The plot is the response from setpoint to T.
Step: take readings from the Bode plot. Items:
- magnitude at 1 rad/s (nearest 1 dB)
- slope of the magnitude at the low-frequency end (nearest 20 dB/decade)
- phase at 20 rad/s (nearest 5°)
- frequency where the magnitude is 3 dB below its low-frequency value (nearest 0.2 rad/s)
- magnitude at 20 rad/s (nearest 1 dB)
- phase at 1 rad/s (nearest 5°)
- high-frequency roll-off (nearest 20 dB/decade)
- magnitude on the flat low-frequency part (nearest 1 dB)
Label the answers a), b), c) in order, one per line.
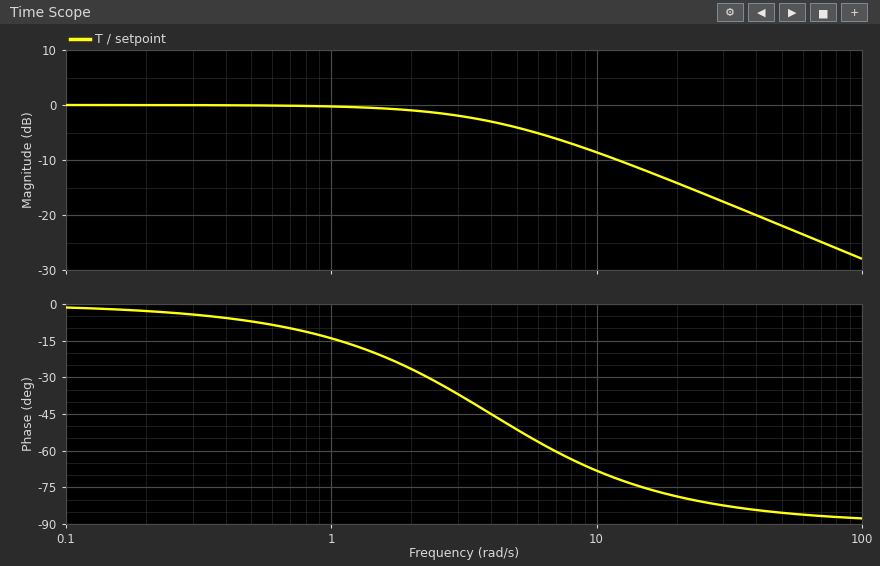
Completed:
a) 0 dB
b) 0 dB/decade
c) -80°
d) 4.0 rad/s
e) -14 dB
f) -15°
g) -20 dB/decade
h) 0 dB
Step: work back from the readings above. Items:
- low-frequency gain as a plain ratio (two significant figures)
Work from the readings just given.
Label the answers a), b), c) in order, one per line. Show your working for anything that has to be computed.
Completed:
a) 10^(0 / 20) = 1.0
